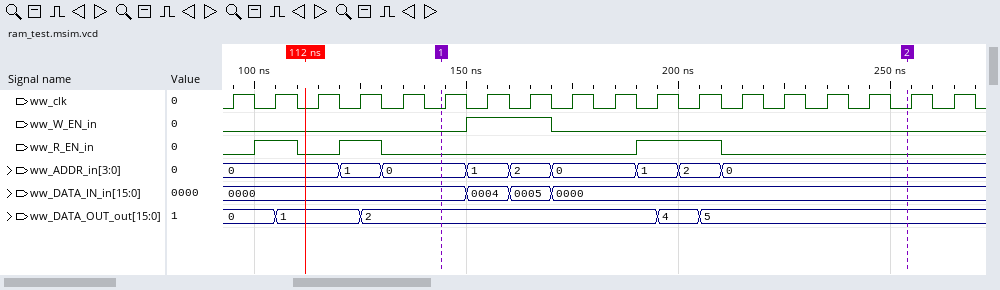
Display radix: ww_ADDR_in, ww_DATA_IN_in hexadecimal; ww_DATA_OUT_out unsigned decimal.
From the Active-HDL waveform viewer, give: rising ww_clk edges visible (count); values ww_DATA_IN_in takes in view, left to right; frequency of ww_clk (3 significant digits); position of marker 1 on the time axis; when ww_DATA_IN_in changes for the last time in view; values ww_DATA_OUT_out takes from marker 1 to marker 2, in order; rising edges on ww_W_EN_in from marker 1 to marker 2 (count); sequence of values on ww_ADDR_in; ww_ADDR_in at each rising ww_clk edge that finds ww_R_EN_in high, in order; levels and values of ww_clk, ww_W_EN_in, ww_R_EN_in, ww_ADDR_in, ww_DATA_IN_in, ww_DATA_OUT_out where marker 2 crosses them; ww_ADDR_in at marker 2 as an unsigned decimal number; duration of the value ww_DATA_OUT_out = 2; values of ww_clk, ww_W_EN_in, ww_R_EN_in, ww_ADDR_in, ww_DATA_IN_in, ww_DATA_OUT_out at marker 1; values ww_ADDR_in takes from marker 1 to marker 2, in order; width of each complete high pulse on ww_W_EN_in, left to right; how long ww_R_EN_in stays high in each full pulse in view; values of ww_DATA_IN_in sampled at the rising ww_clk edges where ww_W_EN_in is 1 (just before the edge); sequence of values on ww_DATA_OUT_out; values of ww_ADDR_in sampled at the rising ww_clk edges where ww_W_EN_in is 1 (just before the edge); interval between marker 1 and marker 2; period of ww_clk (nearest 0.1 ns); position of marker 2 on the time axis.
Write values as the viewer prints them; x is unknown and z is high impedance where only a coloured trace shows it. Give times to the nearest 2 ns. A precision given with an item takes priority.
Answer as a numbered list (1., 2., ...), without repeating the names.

1. 18
2. 0000, 0004, 0005, 0000
3. 100 MHz
4. 144 ns
5. 170 ns
6. 2, 4, 5
7. 1
8. 0, 1, 0, 1, 2, 0, 1, 2, 0
9. 0, 1, 1, 2
10. ww_clk=0, ww_W_EN_in=0, ww_R_EN_in=0, ww_ADDR_in=0, ww_DATA_IN_in=0000, ww_DATA_OUT_out=5
11. 0
12. 70 ns
13. ww_clk=0, ww_W_EN_in=0, ww_R_EN_in=0, ww_ADDR_in=0, ww_DATA_IN_in=0000, ww_DATA_OUT_out=2
14. 0, 1, 2, 0, 1, 2, 0
15. 20 ns
16. 10 ns, 10 ns, 20 ns
17. 0004, 0005
18. 0, 1, 2, 4, 5
19. 1, 2
20. 110 ns
21. 10 ns
22. 254 ns
